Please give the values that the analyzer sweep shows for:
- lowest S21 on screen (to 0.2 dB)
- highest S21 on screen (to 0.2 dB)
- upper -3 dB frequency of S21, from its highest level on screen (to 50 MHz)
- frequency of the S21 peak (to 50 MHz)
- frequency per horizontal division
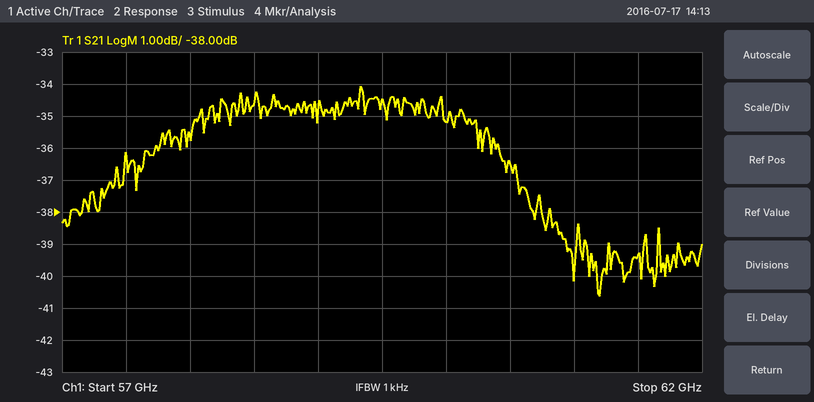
-40.6 dB
-34.0 dB
60.55 GHz
59.35 GHz
500 MHz
